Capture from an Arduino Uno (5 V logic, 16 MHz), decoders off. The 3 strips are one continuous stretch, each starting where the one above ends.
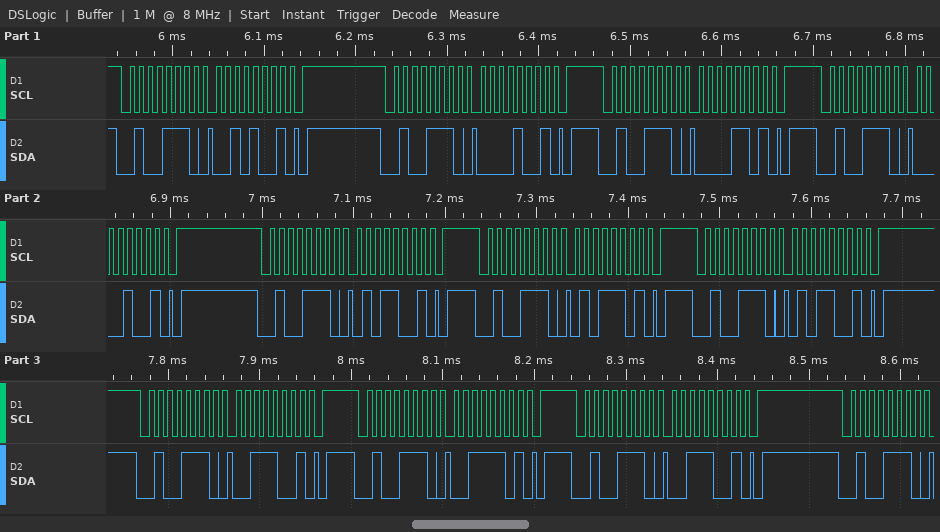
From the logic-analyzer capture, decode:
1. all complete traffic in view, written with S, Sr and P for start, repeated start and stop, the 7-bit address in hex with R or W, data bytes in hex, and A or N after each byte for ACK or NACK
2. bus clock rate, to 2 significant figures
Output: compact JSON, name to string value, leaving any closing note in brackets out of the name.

{"all complete traffic in view, written with S, Sr and P for start, repeated start and stop, the 7-bit address in hex with R or W, data bytes in hex, and A or N after each byte for ACK or NACK": "S 27W A 29 A P S 27W A 09 A P S 27W A 0D A P S 27W A 09 A P S 27W A 59 A P S 27W A 5D A P S 27W A 59 A P S 27W A 39 A P S 27W A 3D A P S 27W A 39 A P S 27W A", "bus clock rate, to 2 significant figures": "100 kHz"}
